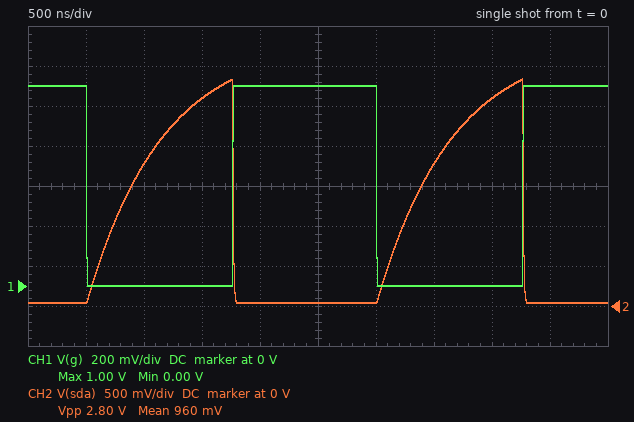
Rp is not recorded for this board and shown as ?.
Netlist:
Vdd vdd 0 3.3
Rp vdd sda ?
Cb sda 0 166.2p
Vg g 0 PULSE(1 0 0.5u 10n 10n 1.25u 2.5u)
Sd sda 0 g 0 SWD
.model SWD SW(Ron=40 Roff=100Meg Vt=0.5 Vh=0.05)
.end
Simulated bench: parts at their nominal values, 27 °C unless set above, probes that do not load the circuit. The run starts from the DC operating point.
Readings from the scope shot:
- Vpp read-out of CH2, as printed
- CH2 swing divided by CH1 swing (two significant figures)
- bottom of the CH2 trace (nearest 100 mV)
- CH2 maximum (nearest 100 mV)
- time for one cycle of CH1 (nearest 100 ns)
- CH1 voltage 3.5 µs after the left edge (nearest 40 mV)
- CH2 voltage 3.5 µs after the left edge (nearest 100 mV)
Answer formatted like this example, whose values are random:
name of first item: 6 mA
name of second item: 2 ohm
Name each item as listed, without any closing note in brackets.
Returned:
Vpp read-out of CH2, as printed: 2.80 V
CH2 swing divided by CH1 swing: 2.8
bottom of the CH2 trace: 0 V
CH2 maximum: 2.8 V
time for one cycle of CH1: 2.5 µs
CH1 voltage 3.5 µs after the left edge: 0 V
CH2 voltage 3.5 µs after the left edge: 1.8 V
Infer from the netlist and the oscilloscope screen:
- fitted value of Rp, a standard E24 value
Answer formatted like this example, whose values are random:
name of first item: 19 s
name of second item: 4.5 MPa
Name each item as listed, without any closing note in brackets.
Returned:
fitted value of Rp, a standard E24 value: 3.9 kΩ
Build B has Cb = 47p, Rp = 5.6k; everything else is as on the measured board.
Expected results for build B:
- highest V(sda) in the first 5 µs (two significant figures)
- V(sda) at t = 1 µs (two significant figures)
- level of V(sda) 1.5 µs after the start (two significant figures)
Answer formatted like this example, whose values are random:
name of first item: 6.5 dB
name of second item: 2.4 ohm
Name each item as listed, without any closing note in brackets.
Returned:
highest V(sda) in the first 5 µs: 3.3 V
V(sda) at t = 1 µs: 2.8 V
level of V(sda) 1.5 µs after the start: 3.2 V
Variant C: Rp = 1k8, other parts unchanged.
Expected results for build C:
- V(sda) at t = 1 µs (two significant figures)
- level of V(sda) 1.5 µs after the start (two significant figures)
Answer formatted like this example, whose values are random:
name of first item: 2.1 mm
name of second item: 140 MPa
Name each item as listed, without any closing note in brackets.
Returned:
V(sda) at t = 1 µs: 2.7 V
level of V(sda) 1.5 µs after the start: 3.2 V
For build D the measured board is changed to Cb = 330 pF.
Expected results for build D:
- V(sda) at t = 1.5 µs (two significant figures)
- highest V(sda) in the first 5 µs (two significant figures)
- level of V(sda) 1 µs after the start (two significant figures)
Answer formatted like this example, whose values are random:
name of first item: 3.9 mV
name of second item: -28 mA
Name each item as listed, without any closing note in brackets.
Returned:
V(sda) at t = 1.5 µs: 1.8 V
highest V(sda) in the first 5 µs: 2.1 V
level of V(sda) 1 µs after the start: 1.1 V
